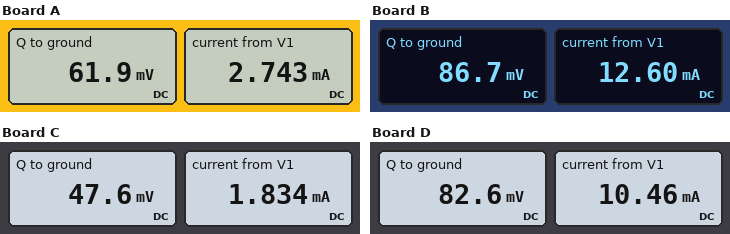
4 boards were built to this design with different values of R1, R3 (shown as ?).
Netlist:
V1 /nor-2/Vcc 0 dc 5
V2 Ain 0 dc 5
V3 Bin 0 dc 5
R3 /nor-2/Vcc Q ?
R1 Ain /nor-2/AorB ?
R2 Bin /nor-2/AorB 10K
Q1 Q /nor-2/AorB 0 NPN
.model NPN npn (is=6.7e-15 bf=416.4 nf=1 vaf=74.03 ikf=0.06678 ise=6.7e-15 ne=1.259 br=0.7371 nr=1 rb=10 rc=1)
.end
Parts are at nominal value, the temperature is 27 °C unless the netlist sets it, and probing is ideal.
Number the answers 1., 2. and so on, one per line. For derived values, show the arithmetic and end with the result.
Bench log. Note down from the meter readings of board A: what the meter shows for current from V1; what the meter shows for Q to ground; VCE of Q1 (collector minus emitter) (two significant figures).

1. 2.743 mA
2. 61.9 mV
3. 61.9 mV = 62 mV
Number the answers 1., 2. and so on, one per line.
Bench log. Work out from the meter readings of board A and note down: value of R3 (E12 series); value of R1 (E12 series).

1. 1.8 kΩ
2. 33 kΩ
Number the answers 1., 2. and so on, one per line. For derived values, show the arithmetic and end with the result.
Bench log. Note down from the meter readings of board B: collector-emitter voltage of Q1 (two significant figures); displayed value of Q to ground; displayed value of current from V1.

1. 86.7 mV = 87 mV
2. 86.7 mV
3. 12.60 mA
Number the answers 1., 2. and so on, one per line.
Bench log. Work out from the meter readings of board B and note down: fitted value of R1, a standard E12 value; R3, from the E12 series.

1. 3.9 kΩ
2. 390 Ω
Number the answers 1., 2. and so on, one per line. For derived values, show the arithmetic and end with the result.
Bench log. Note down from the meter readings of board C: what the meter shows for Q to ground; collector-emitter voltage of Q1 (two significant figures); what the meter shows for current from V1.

1. 47.6 mV
2. 47.6 mV = 48 mV
3. 1.834 mA
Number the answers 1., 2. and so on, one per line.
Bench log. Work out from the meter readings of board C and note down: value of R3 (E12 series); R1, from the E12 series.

1. 2.7 kΩ
2. 12 kΩ
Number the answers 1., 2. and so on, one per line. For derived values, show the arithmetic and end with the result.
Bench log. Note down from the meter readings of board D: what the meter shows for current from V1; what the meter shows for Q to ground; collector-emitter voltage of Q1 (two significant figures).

1. 10.46 mA
2. 82.6 mV
3. 82.6 mV = 83 mV
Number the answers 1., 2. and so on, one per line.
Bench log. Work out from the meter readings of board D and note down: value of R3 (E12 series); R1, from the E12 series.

1. 470 Ω
2. 4.7 kΩ
